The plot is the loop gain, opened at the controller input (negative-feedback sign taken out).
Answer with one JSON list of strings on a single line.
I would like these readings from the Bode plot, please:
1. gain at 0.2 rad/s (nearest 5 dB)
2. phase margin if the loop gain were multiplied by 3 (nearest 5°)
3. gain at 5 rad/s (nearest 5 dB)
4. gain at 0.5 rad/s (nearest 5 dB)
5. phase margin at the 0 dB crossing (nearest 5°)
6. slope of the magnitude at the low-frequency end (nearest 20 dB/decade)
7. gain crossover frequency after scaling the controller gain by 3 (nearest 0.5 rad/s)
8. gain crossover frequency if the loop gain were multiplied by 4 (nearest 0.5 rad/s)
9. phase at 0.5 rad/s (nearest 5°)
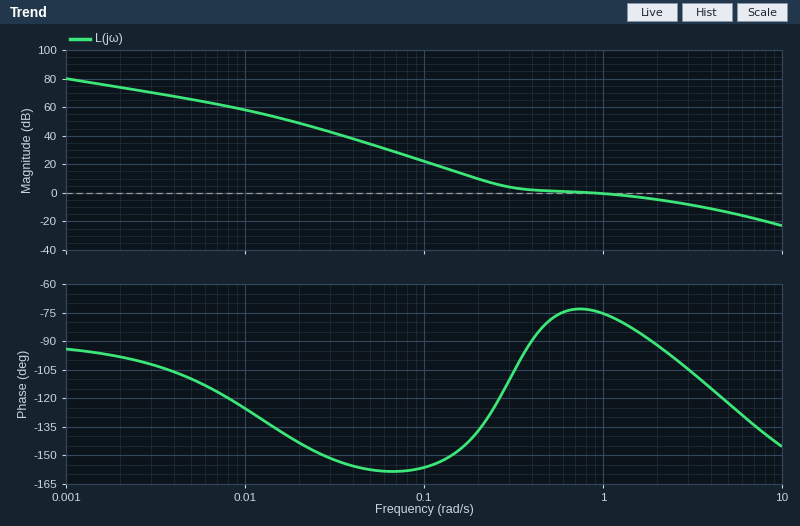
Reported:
["10 dB", "70°", "-15 dB", "0 dB", "105°", "-20 dB/decade", "3.5 rad/s", "4.5 rad/s", "-80°"]
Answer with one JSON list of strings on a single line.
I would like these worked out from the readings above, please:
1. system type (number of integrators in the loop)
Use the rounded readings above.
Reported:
["1"]
